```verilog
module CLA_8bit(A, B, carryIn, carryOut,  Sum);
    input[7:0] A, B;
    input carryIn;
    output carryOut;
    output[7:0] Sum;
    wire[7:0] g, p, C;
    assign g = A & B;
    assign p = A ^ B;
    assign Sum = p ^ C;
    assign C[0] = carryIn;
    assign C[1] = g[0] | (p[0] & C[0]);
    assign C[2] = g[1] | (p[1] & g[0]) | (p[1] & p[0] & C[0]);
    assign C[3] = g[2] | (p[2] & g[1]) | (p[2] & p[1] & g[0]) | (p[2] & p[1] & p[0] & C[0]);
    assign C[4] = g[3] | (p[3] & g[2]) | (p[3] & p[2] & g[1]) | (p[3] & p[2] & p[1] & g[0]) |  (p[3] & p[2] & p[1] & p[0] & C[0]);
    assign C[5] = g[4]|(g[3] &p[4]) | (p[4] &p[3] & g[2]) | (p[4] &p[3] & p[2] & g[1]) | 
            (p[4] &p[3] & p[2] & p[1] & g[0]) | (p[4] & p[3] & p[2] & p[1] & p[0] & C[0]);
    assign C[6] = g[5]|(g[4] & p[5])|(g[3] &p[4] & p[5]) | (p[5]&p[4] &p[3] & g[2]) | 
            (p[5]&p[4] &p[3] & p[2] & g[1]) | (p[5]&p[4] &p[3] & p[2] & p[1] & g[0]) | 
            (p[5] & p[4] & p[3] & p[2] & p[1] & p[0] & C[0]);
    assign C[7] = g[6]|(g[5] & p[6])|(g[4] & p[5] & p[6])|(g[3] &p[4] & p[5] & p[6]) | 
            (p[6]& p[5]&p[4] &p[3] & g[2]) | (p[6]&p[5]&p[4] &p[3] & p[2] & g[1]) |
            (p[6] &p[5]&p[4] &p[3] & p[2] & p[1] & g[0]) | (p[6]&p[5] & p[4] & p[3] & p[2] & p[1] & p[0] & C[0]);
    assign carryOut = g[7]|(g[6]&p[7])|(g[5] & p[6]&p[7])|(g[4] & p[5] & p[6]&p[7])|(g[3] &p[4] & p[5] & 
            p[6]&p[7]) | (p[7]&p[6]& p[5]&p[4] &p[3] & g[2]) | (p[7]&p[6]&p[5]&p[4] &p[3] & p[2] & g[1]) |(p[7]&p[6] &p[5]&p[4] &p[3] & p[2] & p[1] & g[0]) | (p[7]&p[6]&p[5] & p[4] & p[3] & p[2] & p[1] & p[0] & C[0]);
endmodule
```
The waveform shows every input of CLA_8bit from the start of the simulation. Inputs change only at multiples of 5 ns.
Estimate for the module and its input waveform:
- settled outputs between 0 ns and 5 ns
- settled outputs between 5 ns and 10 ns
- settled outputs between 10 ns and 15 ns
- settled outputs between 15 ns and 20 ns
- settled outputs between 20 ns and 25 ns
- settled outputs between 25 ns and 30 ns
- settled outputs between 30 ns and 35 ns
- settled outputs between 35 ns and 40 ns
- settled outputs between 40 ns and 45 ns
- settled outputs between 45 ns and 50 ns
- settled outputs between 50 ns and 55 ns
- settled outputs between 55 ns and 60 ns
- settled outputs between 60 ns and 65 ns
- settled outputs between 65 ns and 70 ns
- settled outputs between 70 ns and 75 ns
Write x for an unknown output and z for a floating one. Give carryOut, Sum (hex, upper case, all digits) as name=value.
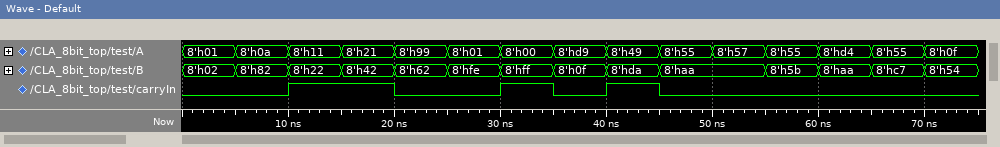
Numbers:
carryOut=0, Sum=03
carryOut=0, Sum=8C
carryOut=0, Sum=34
carryOut=0, Sum=64
carryOut=0, Sum=FB
carryOut=0, Sum=FF
carryOut=1, Sum=00
carryOut=0, Sum=E8
carryOut=1, Sum=24
carryOut=0, Sum=FF
carryOut=1, Sum=01
carryOut=0, Sum=B0
carryOut=1, Sum=7E
carryOut=1, Sum=1C
carryOut=0, Sum=63
